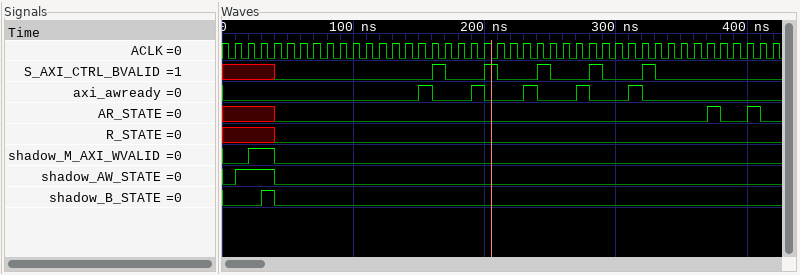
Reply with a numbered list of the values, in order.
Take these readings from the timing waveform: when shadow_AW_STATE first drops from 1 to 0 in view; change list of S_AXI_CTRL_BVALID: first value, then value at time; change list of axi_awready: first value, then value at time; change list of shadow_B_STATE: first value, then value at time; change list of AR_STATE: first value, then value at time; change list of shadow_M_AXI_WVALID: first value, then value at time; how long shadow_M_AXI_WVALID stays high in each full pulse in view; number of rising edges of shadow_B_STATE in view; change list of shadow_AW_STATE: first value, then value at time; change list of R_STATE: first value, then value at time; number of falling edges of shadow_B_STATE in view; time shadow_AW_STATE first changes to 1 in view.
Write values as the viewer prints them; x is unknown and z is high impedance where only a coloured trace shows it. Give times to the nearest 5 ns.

1. 40 ns
2. x, 0 at 40 ns, 1 at 160 ns, 0 at 170 ns, 1 at 200 ns, 0 at 210 ns, 1 at 240 ns, 0 at 250 ns, 1 at 280 ns, 0 at 290 ns, 1 at 320 ns, 0 at 330 ns
3. 0, 1 at 150 ns, 0 at 160 ns, 1 at 190 ns, 0 at 200 ns, 1 at 230 ns, 0 at 240 ns, 1 at 270 ns, 0 at 280 ns, 1 at 310 ns, 0 at 320 ns
4. 0, 1 at 30 ns, 0 at 40 ns
5. x, 0 at 40 ns, 1 at 370 ns, 0 at 380 ns, 1 at 400 ns, 0 at 410 ns
6. 0, 1 at 20 ns, 0 at 40 ns
7. 20 ns
8. 1
9. 0, 1 at 10 ns, 0 at 40 ns
10. x, 0 at 40 ns
11. 1
12. 10 ns
